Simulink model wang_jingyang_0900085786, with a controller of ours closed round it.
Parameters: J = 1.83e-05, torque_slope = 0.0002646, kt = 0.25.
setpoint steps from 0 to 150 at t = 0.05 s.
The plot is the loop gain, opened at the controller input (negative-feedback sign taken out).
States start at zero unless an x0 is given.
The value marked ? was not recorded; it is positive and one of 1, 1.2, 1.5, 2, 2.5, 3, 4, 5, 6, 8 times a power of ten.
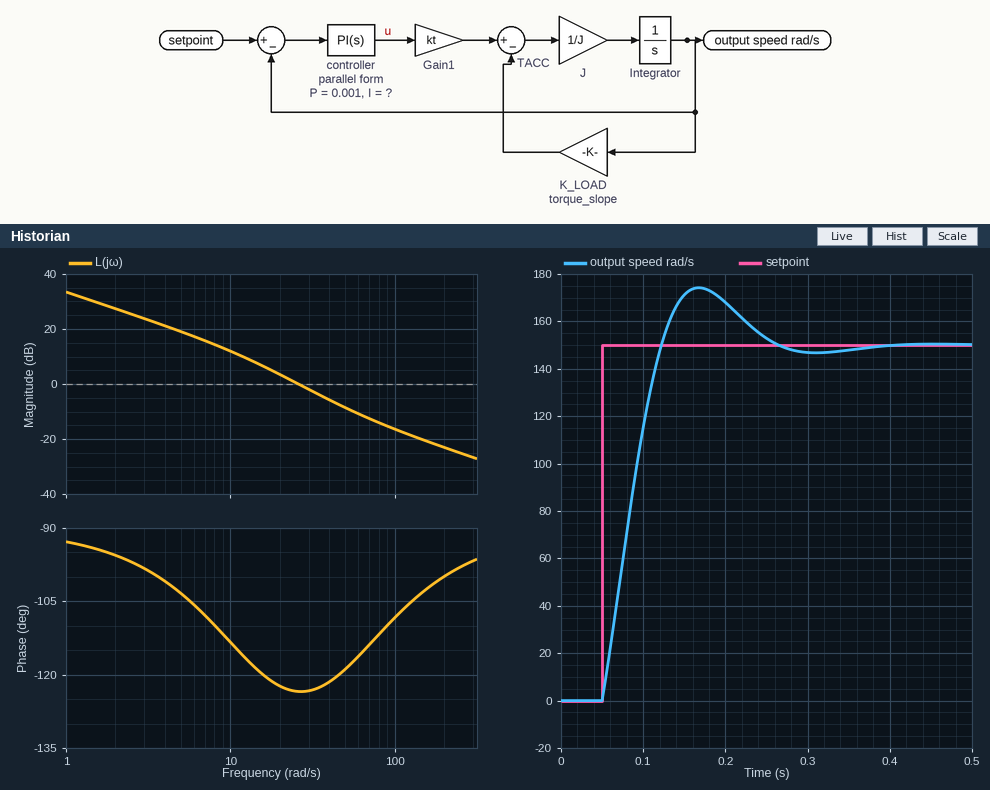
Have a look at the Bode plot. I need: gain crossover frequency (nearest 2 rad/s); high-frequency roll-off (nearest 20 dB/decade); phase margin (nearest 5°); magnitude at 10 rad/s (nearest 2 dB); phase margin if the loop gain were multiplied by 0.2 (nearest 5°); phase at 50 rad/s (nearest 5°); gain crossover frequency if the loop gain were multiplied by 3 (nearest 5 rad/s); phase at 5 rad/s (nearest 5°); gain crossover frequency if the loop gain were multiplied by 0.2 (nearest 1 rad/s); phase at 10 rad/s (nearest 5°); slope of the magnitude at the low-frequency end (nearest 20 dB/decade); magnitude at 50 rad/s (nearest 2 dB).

26 rad/s
-20 dB/decade
55°
12 dB
70°
-120°
55 rad/s
-105°
8 rad/s
-115°
-20 dB/decade
-8 dB
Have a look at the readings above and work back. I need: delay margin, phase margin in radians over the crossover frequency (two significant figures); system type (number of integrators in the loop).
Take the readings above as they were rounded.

0.037 s
1
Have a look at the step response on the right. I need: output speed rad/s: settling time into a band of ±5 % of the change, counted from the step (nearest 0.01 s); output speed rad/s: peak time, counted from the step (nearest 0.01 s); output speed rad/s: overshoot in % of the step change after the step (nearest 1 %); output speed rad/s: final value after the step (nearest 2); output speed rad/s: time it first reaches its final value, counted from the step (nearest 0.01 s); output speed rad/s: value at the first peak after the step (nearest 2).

0.18 s
0.12 s
16 %
150
0.07 s
174
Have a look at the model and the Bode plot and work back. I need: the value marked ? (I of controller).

0.05
